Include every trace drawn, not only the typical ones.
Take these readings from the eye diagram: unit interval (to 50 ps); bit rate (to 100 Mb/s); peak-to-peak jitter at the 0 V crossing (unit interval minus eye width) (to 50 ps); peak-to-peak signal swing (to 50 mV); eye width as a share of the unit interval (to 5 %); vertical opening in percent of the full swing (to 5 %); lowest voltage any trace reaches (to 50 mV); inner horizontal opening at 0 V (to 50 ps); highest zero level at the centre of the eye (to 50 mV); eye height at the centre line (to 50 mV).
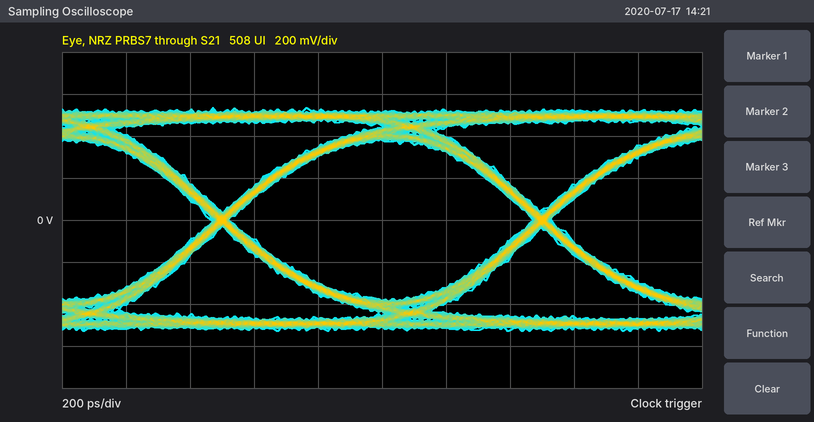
1.00 ns
1.0 Gb/s
50 ps
1.05 V
95 %
70 %
-550 mV
950 ps
-400 mV
750 mV
